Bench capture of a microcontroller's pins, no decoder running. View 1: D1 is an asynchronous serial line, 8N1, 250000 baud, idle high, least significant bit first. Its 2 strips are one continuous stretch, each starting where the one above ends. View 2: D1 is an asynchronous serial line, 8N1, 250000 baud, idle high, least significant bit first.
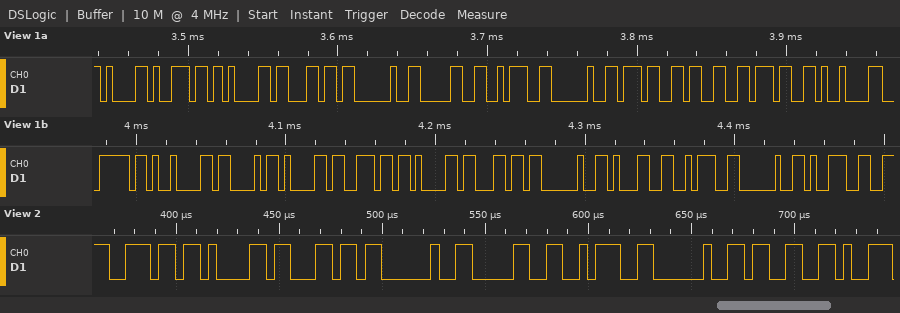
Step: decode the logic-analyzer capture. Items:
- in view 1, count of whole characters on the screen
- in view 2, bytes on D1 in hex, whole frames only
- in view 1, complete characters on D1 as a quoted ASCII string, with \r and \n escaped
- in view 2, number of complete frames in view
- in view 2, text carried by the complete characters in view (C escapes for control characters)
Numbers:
24
0x6E 0x61 0x6C 0x20 0x30 0x3A 0x20 0x33
"anal 0: 737\t|\tCanal 1: 9"
8
"nal 0: 3"
